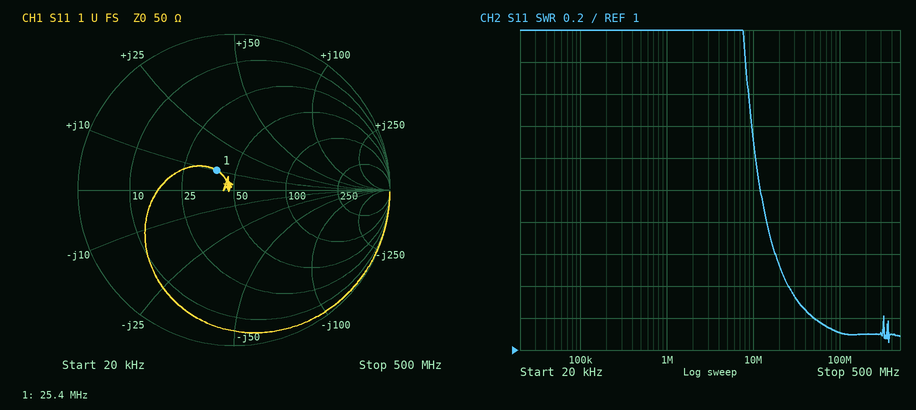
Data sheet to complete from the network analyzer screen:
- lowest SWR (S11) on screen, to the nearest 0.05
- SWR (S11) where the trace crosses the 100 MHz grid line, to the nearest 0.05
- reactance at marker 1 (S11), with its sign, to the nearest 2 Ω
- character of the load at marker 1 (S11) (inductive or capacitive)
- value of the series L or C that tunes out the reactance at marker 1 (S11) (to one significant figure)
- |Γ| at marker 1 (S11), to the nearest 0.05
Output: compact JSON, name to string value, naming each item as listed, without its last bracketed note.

{"lowest SWR (S11) on screen, to the nearest 0.05": "1.05", "SWR (S11) where the trace crosses the 100 MHz grid line, to the nearest 0.05": "1.10", "reactance at marker 1 (S11), with its sign, to the nearest 2 Ω": "+10 Ω", "character of the load at marker 1 (S11)": "inductive", "value of the series L or C that tunes out the reactance at marker 1 (S11)": "600 pF", "|Γ| at marker 1 (S11), to the nearest 0.05": "0.15"}
